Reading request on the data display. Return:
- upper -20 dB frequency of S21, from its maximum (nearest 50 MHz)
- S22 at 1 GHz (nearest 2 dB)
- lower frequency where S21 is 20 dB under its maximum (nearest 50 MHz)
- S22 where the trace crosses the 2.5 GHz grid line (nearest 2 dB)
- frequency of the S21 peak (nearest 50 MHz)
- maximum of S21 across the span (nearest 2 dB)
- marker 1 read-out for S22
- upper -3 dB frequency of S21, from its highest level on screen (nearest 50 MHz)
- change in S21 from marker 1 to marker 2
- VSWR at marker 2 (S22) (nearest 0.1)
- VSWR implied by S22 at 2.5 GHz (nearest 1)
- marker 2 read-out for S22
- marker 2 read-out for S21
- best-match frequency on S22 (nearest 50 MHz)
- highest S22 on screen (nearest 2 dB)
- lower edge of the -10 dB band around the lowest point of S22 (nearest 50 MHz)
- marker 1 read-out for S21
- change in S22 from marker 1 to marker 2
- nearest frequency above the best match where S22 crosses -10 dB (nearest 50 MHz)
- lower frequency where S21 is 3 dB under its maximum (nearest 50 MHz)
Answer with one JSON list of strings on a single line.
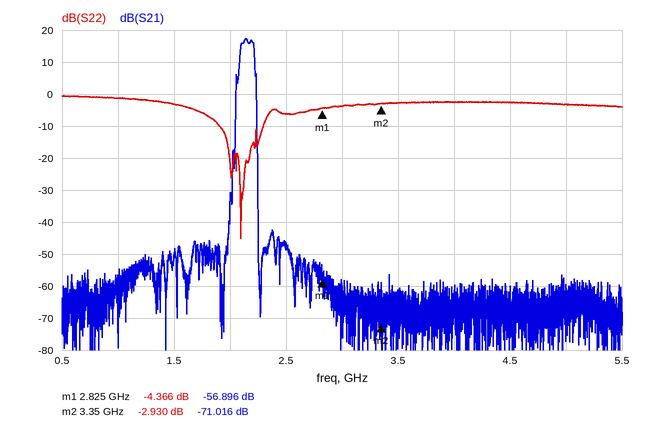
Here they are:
["2.25 GHz", "-2 dB", "2.05 GHz", "-6 dB", "2.15 GHz", "18 dB", "-4.366 dB", "2.20 GHz", "-14.120 dB", "6.0", "3", "-2.930 dB", "-71.016 dB", "2.10 GHz", "0 dB", "1.90 GHz", "-56.896 dB", "1.436 dB", "2.30 GHz", "2.10 GHz"]
